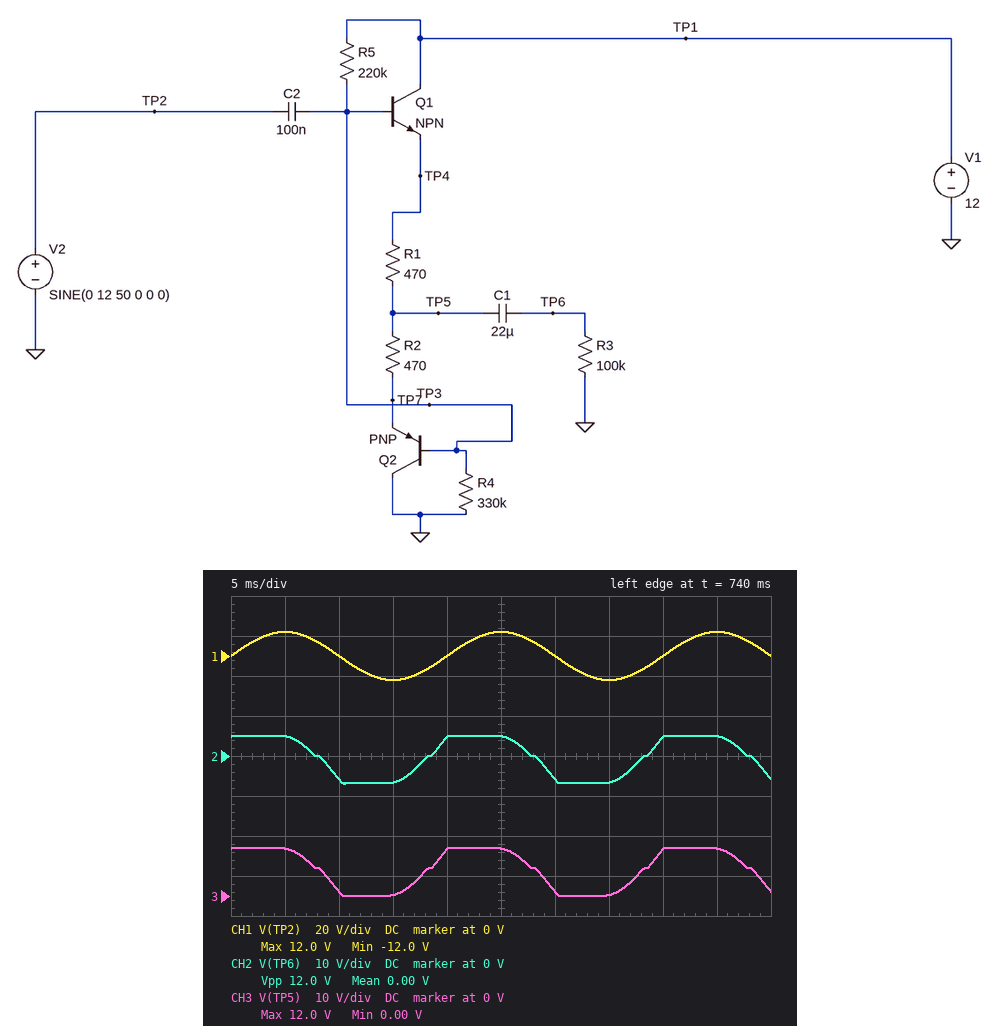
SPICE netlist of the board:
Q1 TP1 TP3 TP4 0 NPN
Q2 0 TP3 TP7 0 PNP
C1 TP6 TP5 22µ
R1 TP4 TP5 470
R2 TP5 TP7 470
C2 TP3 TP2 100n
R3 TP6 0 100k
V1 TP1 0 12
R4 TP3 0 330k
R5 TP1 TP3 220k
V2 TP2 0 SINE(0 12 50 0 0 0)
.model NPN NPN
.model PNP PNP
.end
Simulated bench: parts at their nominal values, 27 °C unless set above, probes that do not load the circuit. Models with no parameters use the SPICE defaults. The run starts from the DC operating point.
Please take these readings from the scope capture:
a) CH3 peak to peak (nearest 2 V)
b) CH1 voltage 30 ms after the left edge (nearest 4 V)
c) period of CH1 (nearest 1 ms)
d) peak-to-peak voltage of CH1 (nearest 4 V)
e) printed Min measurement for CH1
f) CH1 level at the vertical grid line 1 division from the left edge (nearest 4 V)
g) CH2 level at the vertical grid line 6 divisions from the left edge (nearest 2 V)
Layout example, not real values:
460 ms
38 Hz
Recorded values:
12 V
0 V
20 ms
24 V
-12.0 V
12 V
-6 V
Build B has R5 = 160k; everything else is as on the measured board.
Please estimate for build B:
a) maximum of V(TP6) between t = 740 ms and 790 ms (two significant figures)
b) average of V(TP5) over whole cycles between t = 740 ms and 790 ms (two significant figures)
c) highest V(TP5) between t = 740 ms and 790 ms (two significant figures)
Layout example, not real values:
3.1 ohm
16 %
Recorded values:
4.4 V
6.3 V
12 V
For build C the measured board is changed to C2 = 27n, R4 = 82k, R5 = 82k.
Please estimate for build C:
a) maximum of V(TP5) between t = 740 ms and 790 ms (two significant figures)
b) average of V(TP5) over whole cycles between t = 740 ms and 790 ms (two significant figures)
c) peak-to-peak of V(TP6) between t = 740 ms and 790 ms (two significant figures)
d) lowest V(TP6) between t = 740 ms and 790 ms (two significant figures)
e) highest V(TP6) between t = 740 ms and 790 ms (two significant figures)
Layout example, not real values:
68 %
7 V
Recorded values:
9.2 V
6.0 V
6.5 V
-3.2 V
3.2 V
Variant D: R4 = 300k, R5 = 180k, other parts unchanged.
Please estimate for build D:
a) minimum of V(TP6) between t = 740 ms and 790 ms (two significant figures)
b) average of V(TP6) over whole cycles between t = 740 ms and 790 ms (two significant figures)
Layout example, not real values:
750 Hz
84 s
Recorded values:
-7.1 V
-910 mV
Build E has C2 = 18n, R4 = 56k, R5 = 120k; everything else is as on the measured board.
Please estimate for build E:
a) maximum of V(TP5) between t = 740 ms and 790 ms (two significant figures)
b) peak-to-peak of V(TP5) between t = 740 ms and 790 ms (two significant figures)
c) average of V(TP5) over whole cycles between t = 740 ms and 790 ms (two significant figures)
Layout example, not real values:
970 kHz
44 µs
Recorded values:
5.7 V
3.7 V
3.8 V
